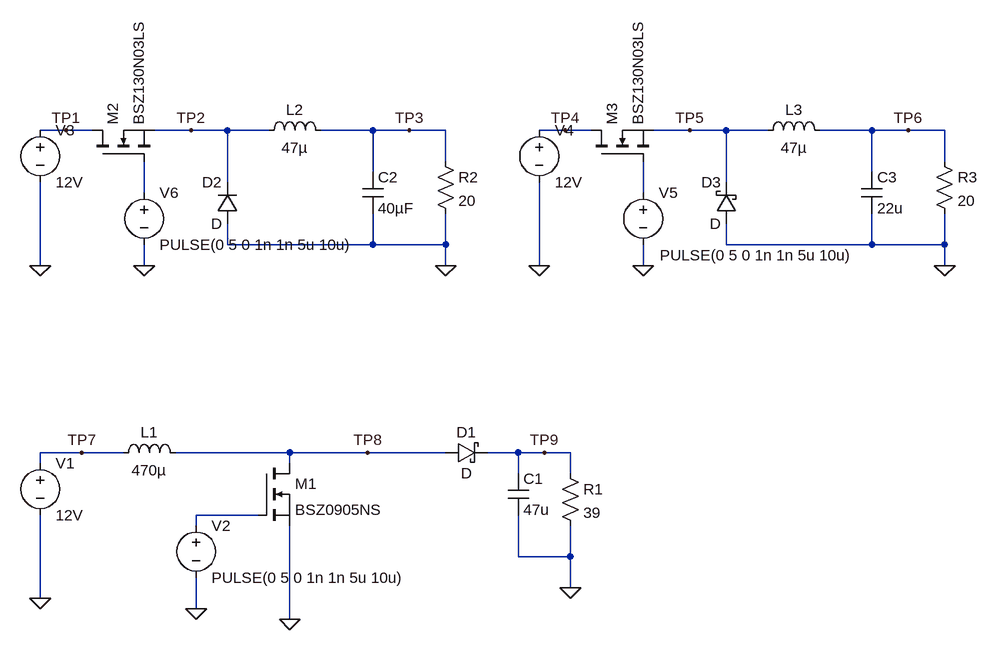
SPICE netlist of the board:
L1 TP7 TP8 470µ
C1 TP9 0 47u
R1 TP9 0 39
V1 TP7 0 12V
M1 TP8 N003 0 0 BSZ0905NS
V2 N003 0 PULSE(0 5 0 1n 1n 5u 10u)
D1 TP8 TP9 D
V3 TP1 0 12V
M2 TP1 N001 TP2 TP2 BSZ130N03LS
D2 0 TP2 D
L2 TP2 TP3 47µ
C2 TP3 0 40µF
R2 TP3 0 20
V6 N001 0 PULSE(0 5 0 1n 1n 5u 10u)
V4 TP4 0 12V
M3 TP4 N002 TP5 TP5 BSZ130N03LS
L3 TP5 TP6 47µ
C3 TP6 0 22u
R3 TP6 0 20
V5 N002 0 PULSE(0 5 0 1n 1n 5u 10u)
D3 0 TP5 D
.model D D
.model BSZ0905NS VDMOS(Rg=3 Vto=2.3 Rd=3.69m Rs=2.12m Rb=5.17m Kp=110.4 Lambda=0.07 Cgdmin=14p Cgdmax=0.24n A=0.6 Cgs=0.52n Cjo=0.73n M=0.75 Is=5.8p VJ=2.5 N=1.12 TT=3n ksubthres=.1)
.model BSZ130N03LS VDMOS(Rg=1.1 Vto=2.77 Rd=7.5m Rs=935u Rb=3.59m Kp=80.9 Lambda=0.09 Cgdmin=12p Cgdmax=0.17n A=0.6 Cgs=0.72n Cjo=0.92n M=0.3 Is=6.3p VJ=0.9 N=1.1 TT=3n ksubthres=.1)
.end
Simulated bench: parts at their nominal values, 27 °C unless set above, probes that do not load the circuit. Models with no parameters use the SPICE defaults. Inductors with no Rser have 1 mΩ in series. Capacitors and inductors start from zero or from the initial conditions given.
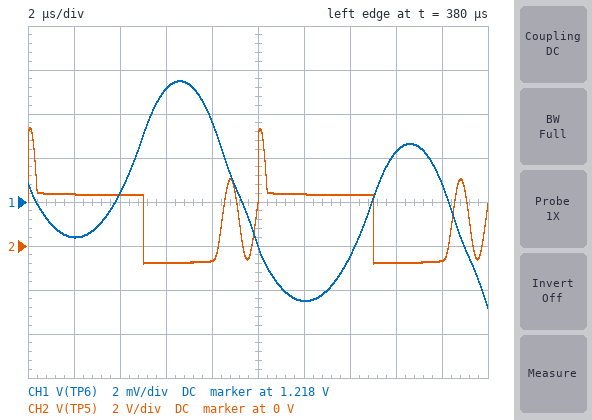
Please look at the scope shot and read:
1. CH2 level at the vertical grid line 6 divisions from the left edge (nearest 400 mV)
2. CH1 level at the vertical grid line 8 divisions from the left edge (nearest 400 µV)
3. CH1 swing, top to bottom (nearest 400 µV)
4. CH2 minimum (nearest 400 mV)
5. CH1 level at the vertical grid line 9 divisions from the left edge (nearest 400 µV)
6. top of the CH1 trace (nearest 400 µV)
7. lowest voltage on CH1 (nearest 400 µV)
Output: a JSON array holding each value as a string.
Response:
["2.4 V", "1.2204 V", "10.4 mV", "-800 mV", "1.2188 V", "1.2236 V", "1.2132 V"]
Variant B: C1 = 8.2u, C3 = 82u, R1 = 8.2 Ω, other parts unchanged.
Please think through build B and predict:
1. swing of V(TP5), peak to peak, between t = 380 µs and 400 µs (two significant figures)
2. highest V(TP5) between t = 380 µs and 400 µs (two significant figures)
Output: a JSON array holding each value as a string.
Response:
["6.9 V", "6.1 V"]
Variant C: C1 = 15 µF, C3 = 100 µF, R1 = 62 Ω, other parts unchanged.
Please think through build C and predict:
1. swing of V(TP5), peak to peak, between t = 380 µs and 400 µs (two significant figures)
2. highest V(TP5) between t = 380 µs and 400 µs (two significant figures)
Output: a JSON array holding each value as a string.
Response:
["6.9 V", "6.1 V"]
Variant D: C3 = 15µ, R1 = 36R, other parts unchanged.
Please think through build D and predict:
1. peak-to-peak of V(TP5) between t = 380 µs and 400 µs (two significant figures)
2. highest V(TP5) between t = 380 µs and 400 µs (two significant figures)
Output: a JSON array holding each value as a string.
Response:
["5.7 V", "4.9 V"]
